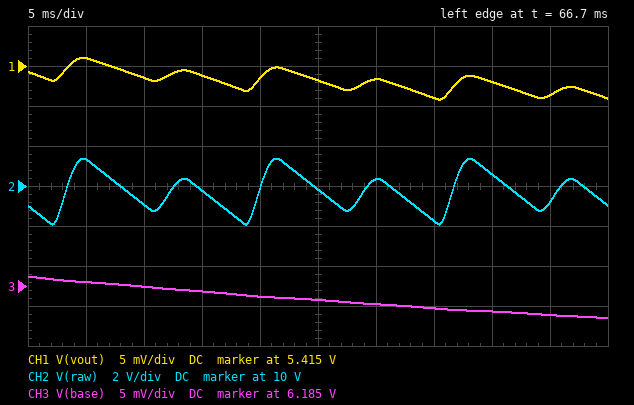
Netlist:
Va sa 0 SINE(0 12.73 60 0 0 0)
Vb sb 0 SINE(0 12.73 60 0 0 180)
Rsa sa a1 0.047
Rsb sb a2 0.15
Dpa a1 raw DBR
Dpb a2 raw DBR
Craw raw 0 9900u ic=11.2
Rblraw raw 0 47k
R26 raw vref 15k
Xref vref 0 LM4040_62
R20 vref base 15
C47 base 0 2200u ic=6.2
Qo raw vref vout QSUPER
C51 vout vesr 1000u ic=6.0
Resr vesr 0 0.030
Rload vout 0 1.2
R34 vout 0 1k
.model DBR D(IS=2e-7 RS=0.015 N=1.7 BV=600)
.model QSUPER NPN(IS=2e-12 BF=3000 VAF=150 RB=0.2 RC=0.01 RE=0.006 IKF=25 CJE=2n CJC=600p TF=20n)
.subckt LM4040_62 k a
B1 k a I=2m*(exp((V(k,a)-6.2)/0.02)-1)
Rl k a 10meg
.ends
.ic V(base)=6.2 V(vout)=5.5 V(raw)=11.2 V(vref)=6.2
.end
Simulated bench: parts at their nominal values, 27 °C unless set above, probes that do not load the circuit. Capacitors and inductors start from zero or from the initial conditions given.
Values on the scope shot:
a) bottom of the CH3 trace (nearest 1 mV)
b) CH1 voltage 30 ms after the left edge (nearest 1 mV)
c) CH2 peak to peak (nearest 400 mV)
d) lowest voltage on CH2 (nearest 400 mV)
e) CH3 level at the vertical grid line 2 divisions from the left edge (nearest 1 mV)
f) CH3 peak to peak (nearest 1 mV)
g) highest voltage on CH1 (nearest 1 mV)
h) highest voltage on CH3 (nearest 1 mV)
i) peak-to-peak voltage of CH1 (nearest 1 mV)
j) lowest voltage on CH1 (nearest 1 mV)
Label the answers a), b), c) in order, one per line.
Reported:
a) 6.181 V
b) 5.413 V
c) 3.2 V
d) 8.0 V
e) 6.185 V
f) 5 mV
g) 5.416 V
h) 6.186 V
i) 5 mV
j) 5.411 V
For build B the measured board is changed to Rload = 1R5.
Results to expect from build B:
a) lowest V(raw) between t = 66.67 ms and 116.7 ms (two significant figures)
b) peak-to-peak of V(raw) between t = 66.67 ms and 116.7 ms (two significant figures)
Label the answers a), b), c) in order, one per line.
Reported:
a) 8.7 V
b) 2.8 V
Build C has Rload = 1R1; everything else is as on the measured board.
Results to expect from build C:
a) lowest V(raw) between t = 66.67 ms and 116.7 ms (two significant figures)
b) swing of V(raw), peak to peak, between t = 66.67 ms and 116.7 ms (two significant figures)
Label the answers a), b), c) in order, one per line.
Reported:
a) 7.8 V
b) 3.5 V
